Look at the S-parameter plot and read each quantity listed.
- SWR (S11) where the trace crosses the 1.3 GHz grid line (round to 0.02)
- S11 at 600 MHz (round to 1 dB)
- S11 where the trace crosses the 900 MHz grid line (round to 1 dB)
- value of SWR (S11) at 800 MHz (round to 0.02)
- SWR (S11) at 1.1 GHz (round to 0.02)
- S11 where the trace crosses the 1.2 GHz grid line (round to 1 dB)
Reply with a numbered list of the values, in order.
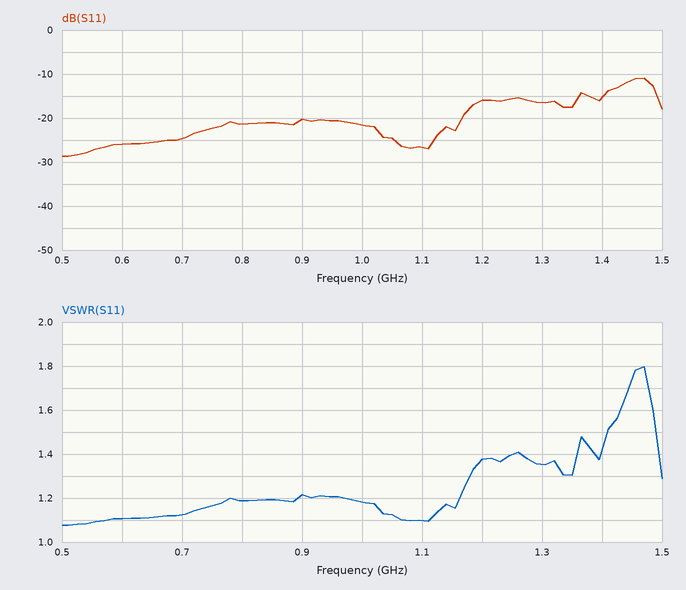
1. 1.36
2. -26 dB
3. -20 dB
4. 1.18
5. 1.10
6. -16 dB
